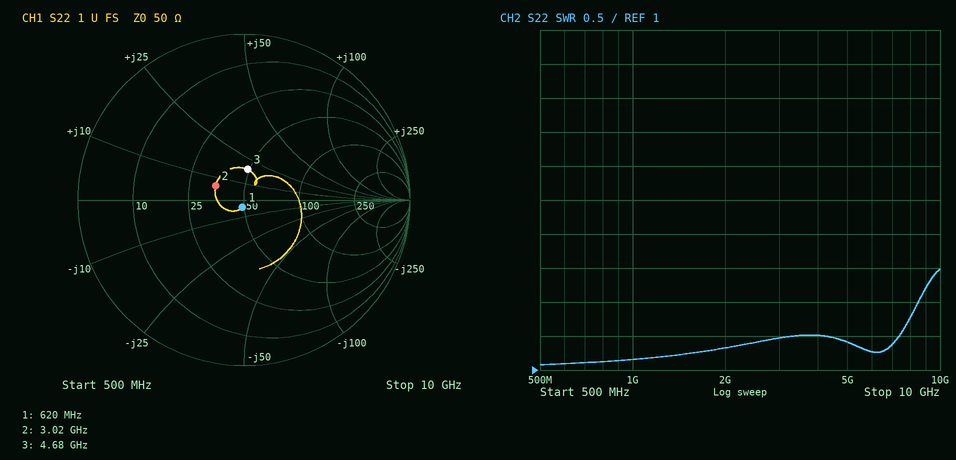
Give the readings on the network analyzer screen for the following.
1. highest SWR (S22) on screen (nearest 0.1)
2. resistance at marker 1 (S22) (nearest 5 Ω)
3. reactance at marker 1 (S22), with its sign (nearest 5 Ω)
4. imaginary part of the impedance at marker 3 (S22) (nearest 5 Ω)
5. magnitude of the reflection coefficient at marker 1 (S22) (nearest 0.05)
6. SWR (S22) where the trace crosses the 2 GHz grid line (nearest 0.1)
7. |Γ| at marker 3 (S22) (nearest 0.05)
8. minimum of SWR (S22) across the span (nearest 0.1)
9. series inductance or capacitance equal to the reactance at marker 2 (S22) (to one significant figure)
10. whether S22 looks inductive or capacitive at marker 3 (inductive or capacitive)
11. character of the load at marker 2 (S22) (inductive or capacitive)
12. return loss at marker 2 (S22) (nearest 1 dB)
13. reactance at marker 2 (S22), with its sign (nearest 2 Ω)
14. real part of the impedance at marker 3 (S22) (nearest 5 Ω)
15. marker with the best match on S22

2.5
50 Ω
-5 Ω
+20 Ω
0.05
1.3
0.20
1.1
300 pH
inductive
inductive
14 dB
+6 Ω
50 Ω
marker 1
